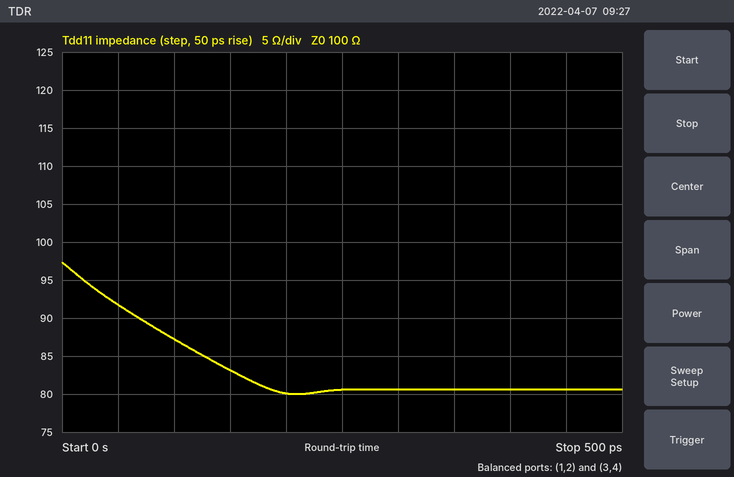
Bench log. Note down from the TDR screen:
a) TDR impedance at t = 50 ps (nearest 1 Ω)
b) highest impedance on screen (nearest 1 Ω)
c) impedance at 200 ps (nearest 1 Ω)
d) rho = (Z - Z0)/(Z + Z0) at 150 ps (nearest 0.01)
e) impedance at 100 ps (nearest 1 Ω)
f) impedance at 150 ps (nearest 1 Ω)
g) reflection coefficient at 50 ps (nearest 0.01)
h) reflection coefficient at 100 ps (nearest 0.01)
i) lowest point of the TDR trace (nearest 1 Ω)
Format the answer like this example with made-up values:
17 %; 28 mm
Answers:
92 Ω; 97 Ω; 80 Ω; -0.09; 87 Ω; 83 Ω; -0.04; -0.07; 80 Ω
